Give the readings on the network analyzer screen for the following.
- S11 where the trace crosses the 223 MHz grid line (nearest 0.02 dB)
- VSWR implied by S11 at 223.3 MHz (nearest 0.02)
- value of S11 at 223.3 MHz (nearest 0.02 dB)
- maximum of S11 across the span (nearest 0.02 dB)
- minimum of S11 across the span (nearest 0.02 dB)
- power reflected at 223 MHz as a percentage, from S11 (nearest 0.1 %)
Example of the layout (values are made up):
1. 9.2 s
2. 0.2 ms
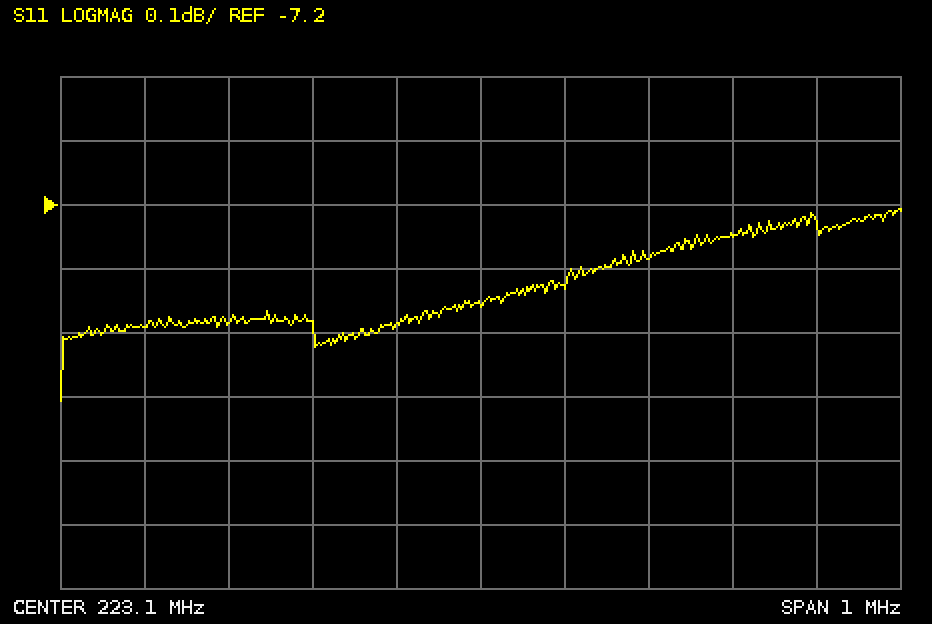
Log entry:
1. -7.38 dB
2. 2.52
3. -7.28 dB
4. -7.20 dB
5. -7.50 dB
6. 18.3 %
